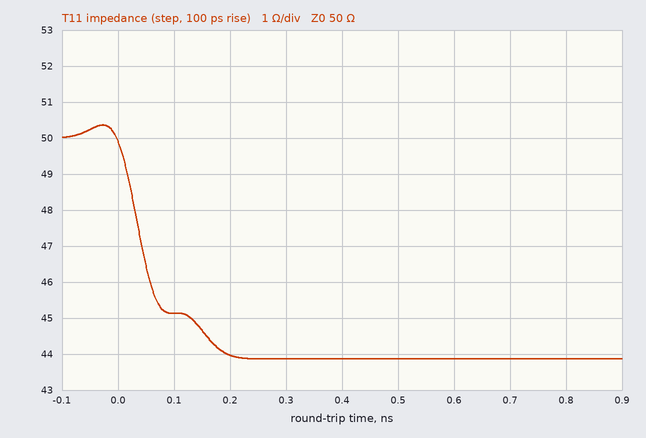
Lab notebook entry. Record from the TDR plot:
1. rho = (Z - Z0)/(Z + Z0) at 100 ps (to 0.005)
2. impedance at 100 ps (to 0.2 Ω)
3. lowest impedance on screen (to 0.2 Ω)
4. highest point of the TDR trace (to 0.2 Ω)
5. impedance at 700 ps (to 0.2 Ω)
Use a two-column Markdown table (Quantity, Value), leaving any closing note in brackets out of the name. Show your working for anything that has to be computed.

| Quantity | Value |
|---|---|
| rho = (Z - Z0)/(Z + Z0) at 100 ps | (45.2 − 50)/(45.2 + 50) ≈ -0.050 |
| impedance at 100 ps | 45.2 Ω |
| lowest impedance on screen | 43.8 Ω |
| highest point of the TDR trace | 50.4 Ω |
| impedance at 700 ps | 43.8 Ω |
